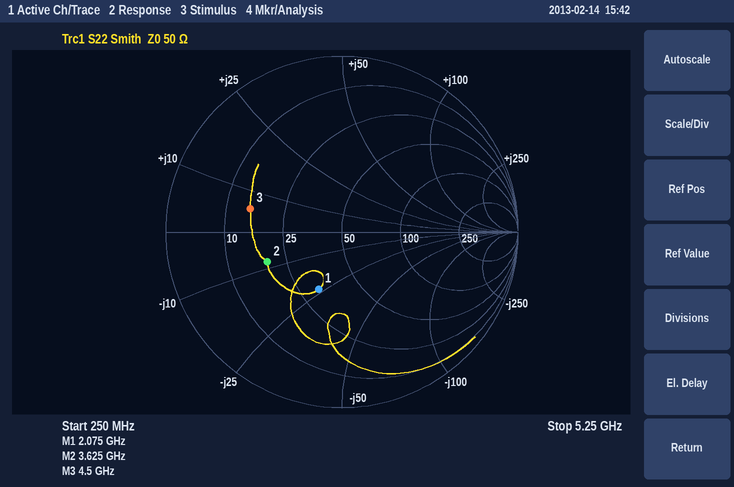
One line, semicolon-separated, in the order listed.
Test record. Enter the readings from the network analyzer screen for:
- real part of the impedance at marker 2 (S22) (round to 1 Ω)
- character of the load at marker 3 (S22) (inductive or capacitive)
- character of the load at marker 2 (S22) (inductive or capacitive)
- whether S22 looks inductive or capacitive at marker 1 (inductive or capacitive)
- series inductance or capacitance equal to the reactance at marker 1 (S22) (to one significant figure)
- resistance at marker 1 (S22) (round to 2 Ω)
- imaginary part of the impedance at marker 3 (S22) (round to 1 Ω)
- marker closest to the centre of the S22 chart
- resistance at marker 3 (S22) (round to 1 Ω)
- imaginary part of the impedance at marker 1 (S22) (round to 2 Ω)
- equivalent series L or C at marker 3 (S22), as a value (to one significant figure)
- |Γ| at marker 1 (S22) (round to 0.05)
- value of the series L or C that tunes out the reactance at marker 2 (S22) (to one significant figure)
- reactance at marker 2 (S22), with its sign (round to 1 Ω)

19 Ω; inductive; capacitive; capacitive; 3 pF; 32 Ω; +6 Ω; marker 1; 15 Ω; -24 Ω; 200 pH; 0.35; 400 pH; -8 Ω
